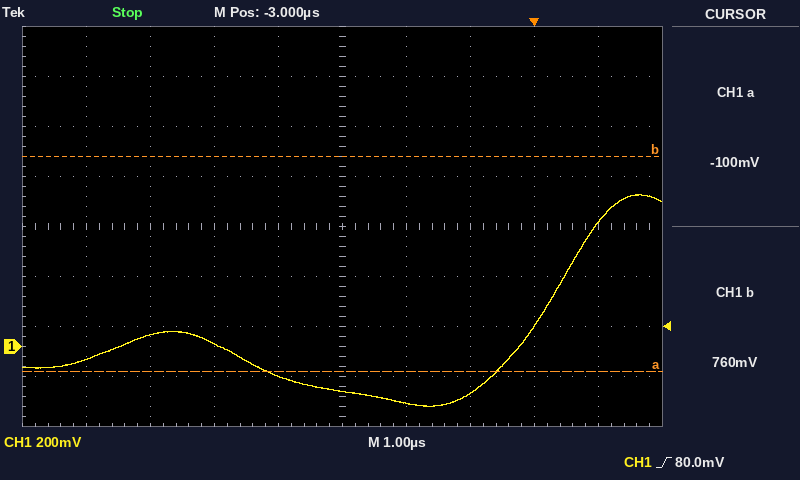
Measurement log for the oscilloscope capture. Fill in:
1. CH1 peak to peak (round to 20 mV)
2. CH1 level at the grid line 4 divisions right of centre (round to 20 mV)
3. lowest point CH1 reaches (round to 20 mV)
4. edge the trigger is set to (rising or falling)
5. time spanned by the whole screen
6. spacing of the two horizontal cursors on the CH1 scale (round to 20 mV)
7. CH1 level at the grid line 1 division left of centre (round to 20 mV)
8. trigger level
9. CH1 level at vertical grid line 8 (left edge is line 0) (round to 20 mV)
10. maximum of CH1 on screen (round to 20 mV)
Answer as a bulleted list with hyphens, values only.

- 840 mV
- 500 mV
- -240 mV
- rising
- 10 µs
- 860 mV
- -120 mV
- 80.0 mV
- 80 mV
- 600 mV
